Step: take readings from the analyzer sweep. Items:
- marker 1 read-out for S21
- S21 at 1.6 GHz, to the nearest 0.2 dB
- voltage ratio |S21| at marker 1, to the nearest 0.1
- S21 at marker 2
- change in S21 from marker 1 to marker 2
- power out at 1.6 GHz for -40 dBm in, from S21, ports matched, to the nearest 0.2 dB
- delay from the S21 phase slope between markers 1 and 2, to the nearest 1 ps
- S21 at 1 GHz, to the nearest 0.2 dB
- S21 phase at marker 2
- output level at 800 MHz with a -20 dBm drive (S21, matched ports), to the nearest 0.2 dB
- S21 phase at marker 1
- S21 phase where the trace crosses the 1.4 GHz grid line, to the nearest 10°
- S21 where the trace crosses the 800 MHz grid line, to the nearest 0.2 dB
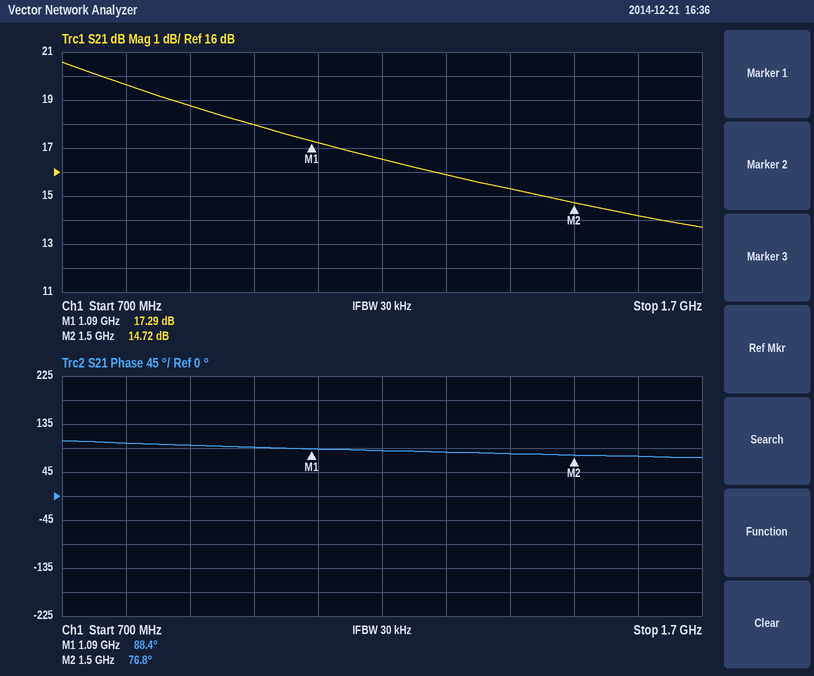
17.29 dB
14.2 dB
7.3
14.72 dB
-2.57 dB
-25.8 dBm
79 ps
18.0 dB
76.8°
-0.4 dBm
88.4°
80°
19.6 dB
